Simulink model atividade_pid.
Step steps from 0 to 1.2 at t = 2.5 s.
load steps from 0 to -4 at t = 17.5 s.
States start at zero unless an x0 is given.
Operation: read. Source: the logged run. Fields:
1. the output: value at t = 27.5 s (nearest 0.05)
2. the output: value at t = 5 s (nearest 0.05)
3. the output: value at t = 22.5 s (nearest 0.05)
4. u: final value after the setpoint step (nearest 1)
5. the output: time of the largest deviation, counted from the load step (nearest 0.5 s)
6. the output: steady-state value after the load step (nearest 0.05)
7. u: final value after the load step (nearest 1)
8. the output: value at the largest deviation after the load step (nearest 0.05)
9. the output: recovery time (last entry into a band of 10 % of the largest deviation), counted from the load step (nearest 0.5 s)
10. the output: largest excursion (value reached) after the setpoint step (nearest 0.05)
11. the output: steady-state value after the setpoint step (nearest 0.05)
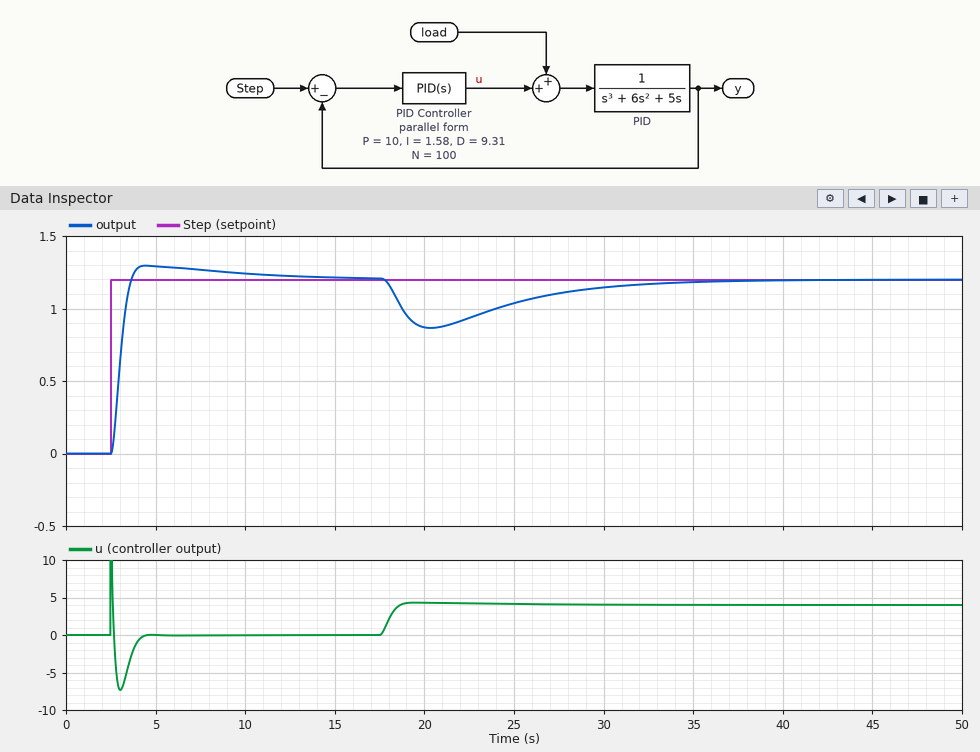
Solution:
1.10
1.30
0.95
0
3.0 s
1.20
4
0.85
14.5 s
1.30
1.20
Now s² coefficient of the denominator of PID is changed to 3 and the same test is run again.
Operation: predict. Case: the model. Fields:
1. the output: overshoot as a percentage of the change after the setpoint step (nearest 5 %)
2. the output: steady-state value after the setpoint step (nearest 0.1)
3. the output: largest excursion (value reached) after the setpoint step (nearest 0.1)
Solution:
15 %
1.2
1.4
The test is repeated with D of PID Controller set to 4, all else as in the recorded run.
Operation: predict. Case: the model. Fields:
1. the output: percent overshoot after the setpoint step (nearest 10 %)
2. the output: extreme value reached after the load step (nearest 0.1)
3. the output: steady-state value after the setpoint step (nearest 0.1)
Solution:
30 %
0.8
1.2
